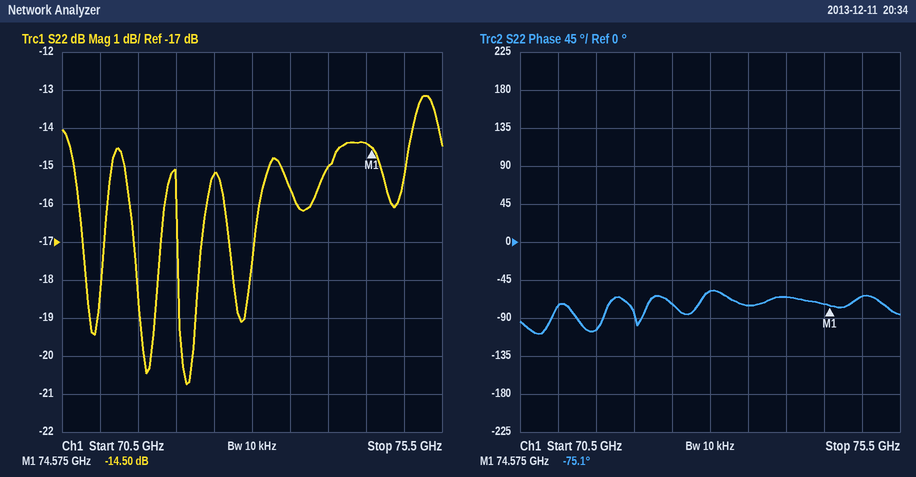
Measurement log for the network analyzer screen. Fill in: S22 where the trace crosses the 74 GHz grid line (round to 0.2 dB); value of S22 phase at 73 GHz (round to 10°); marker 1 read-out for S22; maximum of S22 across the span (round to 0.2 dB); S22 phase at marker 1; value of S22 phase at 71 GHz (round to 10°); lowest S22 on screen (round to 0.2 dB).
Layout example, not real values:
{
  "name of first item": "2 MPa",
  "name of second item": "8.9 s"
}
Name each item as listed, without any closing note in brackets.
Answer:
{
  "S22 where the trace crosses the 74 GHz grid line": "-15.0 dB",
  "value of S22 phase at 73 GHz": "-60°",
  "marker 1 read-out for S22": "-14.50 dB",
  "maximum of S22 across the span": "-13.2 dB",
  "S22 phase at marker 1": "-75.1°",
  "value of S22 phase at 71 GHz": "-80°",
  "lowest S22 on screen": "-20.8 dB"
}
